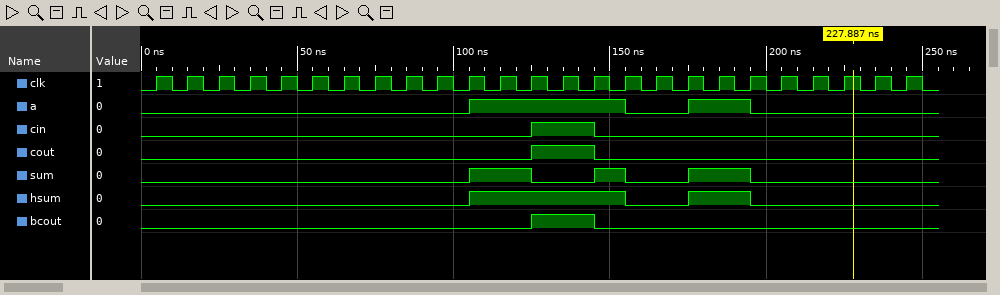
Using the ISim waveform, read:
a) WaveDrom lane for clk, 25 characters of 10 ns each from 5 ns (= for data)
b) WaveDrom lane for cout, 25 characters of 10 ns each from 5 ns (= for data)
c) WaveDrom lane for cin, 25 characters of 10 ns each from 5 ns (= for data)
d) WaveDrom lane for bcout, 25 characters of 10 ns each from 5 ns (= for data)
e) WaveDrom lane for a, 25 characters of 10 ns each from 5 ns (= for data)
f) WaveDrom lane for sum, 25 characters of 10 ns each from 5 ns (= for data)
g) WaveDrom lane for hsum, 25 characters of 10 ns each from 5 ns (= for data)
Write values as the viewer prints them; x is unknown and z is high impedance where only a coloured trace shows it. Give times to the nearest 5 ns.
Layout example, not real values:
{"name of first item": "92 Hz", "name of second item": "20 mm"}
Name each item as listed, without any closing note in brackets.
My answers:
{"WaveDrom lane for clk, 25 characters of 10 ns each from 5 ns": "{name: 'clk', wave: 'p........................'}", "WaveDrom lane for cout, 25 characters of 10 ns each from 5 ns": "{name: 'cout', wave: '0...........1.0..........'}", "WaveDrom lane for cin, 25 characters of 10 ns each from 5 ns": "{name: 'cin', wave: '0...........1.0..........'}", "WaveDrom lane for bcout, 25 characters of 10 ns each from 5 ns": "{name: 'bcout', wave: '0...........1.0..........'}", "WaveDrom lane for a, 25 characters of 10 ns each from 5 ns": "{name: 'a', wave: '0.........1....0.1.0.....'}", "WaveDrom lane for sum, 25 characters of 10 ns each from 5 ns": "{name: 'sum', wave: '0.........1.0.10.1.0.....'}", "WaveDrom lane for hsum, 25 characters of 10 ns each from 5 ns": "{name: 'hsum', wave: '0.........1....0.1.0.....'}"}
